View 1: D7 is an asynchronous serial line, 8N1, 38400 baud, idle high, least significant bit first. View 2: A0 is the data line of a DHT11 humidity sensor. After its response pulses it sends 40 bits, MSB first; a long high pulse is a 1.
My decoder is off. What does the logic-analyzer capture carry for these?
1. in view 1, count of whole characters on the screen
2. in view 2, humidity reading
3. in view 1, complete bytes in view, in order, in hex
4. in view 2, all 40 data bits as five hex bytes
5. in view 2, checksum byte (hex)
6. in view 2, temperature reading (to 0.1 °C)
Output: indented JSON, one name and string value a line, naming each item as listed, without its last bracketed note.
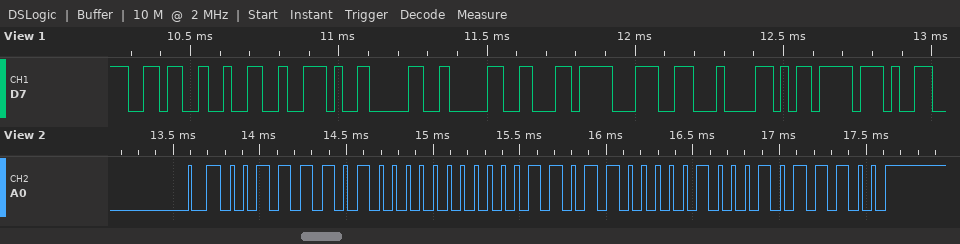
{
  "in view 1, count of whole characters on the screen": "10",
  "in view 2, humidity reading": "61 %",
  "in view 1, complete bytes in view, in order, in hex": "36 32 2E 30 30 EC 9C 84 ED 97",
  "in view 2, all 40 data bits as five hex bytes": "3D 00 1B 04 5C",
  "in view 2, checksum byte": "0x5C",
  "in view 2, temperature reading": "27.4 °C"
}
